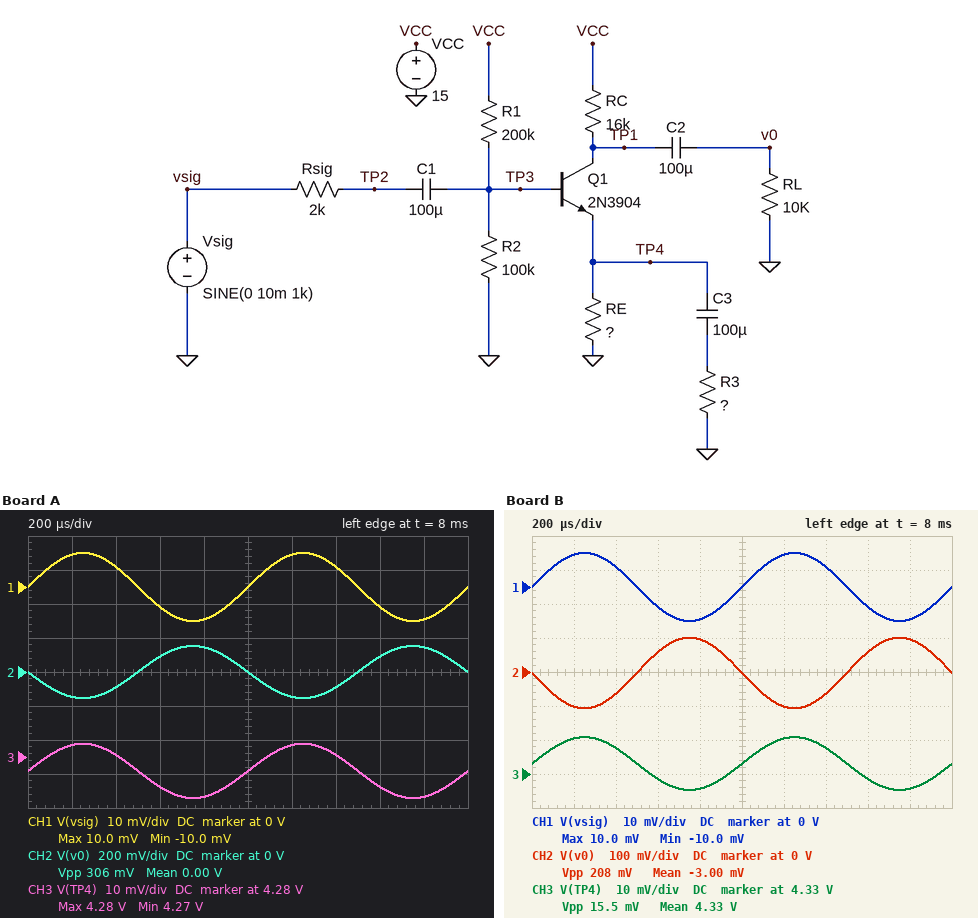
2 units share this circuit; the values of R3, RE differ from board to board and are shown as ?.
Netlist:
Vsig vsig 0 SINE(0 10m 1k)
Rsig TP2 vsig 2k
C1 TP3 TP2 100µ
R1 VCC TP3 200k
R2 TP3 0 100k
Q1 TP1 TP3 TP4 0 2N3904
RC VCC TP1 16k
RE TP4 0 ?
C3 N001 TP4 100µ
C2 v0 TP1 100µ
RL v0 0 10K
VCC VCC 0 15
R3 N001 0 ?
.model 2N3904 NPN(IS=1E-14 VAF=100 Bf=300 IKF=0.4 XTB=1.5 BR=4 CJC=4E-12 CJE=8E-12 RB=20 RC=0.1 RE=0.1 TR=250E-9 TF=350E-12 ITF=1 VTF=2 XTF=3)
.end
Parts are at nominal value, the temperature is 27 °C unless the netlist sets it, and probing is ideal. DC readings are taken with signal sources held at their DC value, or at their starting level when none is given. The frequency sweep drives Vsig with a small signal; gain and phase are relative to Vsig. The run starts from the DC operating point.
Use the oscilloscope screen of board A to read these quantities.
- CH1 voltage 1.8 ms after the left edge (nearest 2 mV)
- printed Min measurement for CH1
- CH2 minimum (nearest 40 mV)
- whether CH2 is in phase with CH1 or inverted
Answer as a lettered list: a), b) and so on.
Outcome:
a) -10 mV
b) -10.0 mV
c) -160 mV
d) inverted
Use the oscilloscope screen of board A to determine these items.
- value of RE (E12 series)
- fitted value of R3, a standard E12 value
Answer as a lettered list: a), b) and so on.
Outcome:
a) 10 kΩ
b) 330 Ω
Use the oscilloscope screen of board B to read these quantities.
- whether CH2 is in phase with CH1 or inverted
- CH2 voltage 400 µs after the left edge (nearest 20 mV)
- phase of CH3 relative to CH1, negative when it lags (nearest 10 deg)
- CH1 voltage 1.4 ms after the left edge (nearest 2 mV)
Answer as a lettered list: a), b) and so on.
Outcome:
a) inverted
b) -60 mV
c) 0 deg
d) 6 mV
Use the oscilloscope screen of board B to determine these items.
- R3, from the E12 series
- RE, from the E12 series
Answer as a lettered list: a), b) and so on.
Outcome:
a) 470 Ω
b) 18 kΩ
